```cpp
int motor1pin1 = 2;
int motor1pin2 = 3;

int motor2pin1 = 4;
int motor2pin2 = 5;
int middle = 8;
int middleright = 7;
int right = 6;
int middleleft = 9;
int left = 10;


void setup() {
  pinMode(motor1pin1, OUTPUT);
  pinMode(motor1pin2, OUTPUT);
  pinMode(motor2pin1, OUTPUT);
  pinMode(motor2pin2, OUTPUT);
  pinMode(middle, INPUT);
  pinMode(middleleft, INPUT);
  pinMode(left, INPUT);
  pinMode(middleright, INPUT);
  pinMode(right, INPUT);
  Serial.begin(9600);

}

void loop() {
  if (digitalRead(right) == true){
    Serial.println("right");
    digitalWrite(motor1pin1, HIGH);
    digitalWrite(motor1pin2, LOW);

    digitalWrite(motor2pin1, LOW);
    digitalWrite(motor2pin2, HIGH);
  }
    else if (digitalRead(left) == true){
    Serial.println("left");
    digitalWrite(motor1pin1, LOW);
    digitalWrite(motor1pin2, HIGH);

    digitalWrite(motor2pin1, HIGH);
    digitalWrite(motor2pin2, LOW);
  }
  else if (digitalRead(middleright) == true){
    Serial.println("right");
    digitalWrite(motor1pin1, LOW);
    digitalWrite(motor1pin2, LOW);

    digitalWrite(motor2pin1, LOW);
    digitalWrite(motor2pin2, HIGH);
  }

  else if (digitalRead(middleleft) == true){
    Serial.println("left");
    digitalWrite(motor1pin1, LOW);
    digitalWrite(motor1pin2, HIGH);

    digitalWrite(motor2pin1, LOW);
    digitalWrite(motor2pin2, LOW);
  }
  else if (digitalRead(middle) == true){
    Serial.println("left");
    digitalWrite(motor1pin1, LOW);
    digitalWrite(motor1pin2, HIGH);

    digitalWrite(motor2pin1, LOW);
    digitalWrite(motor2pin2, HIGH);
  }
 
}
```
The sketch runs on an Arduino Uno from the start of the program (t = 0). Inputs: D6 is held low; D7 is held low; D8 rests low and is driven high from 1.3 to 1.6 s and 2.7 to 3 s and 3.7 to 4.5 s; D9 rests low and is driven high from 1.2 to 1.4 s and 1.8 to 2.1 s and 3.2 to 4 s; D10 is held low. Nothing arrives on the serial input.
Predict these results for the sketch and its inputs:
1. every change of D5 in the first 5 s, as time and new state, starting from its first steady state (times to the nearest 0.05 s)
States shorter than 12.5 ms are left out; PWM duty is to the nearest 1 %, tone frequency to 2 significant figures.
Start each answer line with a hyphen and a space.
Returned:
- 0 s low; 1.4 s high; 1.8 s low; 2.7 s high; 3.2 s low; 4 s high
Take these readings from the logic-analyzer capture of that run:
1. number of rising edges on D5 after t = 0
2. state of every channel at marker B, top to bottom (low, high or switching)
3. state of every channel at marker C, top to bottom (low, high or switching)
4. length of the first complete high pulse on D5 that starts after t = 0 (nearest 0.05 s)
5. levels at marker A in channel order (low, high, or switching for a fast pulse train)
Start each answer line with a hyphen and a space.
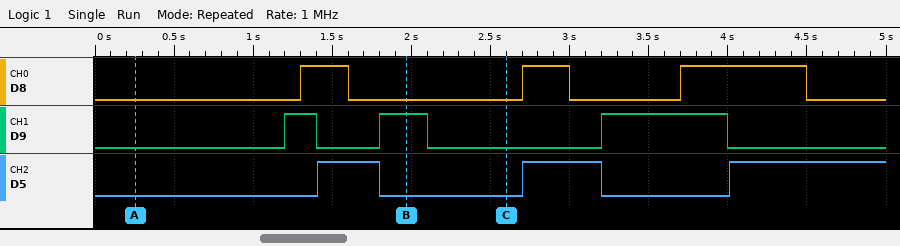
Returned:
- 3
- D8 low, D9 high, D5 low
- D8 low, D9 low, D5 low
- 0.40 s
- D8 low, D9 low, D5 low
